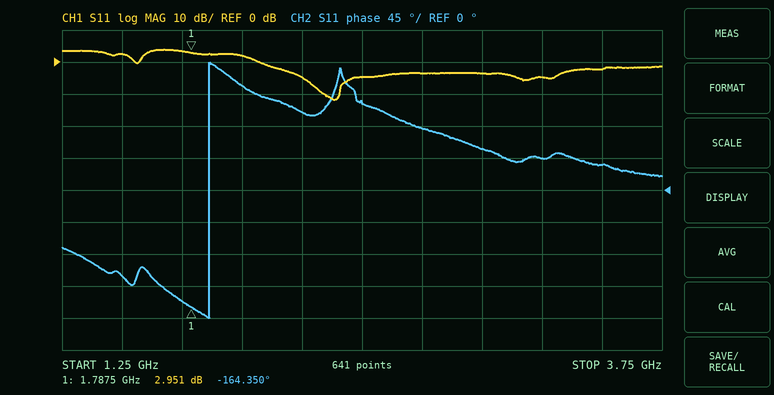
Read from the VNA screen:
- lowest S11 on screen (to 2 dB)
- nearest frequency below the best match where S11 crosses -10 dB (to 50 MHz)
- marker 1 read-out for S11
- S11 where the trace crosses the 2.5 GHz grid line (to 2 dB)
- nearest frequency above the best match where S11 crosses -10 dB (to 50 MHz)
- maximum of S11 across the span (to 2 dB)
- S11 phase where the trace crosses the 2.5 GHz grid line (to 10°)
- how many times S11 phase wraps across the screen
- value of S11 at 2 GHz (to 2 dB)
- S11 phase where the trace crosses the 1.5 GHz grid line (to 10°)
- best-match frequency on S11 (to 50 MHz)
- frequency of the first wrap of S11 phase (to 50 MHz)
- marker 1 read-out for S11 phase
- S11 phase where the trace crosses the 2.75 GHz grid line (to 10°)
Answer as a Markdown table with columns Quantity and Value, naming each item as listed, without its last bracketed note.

| Quantity | Value |
|---|---|
| lowest S11 on screen | -12 dB |
| nearest frequency below the best match where S11 crosses -10 dB | 2.35 GHz |
| marker 1 read-out for S11 | 2.951 dB |
| S11 where the trace crosses the 2.5 GHz grid line | -4 dB |
| nearest frequency above the best match where S11 crosses -10 dB | 2.40 GHz |
| maximum of S11 across the span | 4 dB |
| S11 phase where the trace crosses the 2.5 GHz grid line | 120° |
| how many times S11 phase wraps across the screen | 1 |
| value of S11 at 2 GHz | 2 dB |
| S11 phase where the trace crosses the 1.5 GHz grid line | -120° |
| best-match frequency on S11 | 2.40 GHz |
| frequency of the first wrap of S11 phase | 1.85 GHz |
| marker 1 read-out for S11 phase | -164.350° |
| S11 phase where the trace crosses the 2.75 GHz grid line | 90° |
